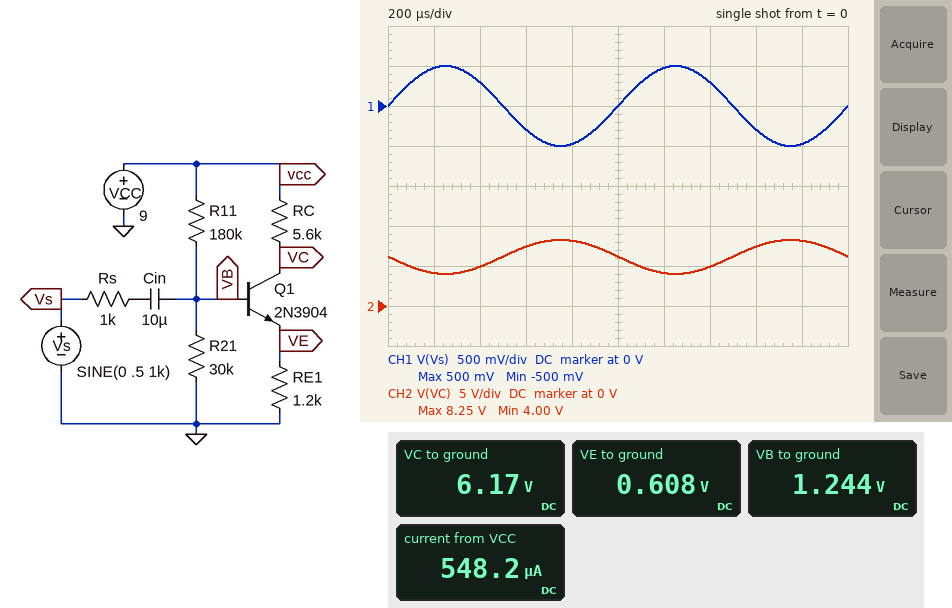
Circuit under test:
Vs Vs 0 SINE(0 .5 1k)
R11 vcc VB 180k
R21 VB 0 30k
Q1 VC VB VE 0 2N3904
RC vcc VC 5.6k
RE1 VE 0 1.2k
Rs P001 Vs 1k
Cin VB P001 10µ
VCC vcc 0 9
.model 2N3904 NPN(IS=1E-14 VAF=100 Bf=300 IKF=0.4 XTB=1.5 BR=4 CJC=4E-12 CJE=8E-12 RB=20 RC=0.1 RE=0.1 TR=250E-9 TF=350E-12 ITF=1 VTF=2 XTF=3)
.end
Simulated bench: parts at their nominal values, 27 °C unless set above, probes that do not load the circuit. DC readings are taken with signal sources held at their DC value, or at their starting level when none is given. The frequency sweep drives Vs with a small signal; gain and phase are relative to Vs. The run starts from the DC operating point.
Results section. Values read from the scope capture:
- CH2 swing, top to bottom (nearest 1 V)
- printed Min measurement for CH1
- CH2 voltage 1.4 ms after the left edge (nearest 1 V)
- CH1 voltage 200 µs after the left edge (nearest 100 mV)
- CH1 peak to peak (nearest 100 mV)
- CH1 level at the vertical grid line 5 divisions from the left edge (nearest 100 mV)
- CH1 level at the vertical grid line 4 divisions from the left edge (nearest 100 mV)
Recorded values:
4 V
-500 mV
5 V
500 mV
1.0 V
0 V
-500 mV
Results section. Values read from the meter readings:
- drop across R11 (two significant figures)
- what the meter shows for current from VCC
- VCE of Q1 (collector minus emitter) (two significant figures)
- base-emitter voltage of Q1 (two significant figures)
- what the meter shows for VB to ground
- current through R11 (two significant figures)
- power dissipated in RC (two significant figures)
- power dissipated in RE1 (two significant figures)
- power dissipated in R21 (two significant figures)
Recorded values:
7.8 V
548.2 µA
5.6 V
640 mV
1.244 V
43 µA
1.4 mW
310 µW
52 µW
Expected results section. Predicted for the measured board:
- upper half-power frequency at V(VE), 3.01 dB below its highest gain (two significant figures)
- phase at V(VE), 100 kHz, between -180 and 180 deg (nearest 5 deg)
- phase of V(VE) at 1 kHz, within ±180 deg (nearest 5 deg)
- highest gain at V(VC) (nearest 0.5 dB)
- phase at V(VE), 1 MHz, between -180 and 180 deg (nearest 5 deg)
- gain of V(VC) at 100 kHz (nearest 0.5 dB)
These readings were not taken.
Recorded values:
9.6 MHz
0 deg
0 deg
12.5 dB
-5 deg
12.5 dB
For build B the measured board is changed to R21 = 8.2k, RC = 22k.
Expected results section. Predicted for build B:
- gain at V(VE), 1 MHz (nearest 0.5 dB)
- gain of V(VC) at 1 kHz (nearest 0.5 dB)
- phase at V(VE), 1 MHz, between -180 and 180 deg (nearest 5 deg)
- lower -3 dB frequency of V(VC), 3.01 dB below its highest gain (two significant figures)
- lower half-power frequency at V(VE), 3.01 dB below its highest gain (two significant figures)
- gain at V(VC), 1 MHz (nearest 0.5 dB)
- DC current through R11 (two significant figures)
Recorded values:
-23.5 dB
-30.0 dB
80 deg
2.5 MHz
7.5 MHz
-13.5 dB
48 µA
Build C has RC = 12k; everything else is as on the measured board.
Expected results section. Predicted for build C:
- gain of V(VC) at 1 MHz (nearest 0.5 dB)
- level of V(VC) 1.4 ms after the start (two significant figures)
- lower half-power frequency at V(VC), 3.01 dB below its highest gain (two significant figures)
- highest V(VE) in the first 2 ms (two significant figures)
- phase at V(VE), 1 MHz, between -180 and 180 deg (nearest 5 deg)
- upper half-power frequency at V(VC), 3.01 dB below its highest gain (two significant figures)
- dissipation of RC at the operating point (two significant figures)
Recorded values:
18.5 dB
900 mV
640 mHz
950 mV
-10 deg
2.6 MHz
3.0 mW
